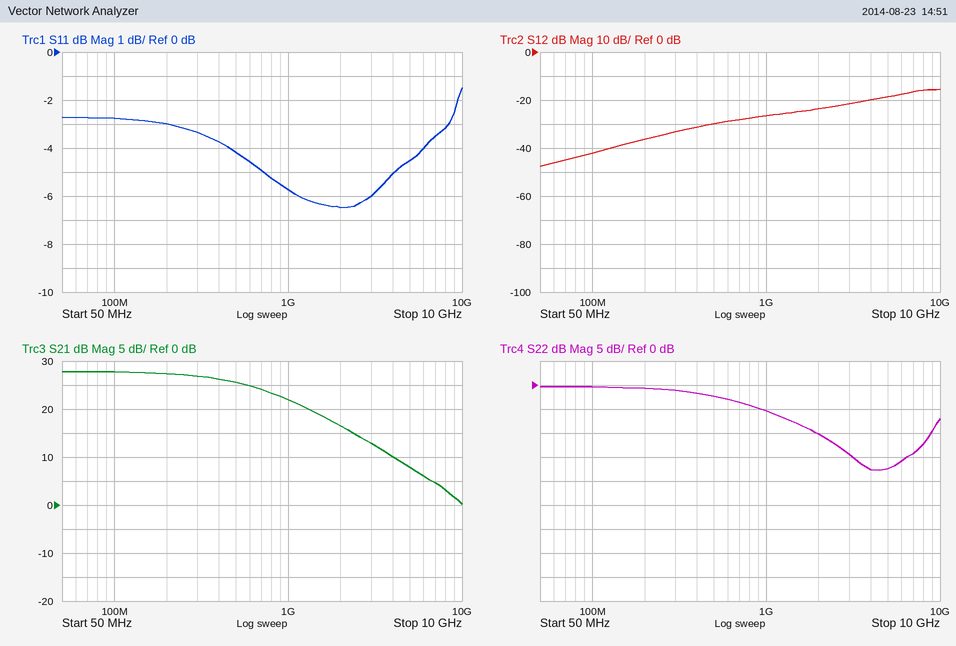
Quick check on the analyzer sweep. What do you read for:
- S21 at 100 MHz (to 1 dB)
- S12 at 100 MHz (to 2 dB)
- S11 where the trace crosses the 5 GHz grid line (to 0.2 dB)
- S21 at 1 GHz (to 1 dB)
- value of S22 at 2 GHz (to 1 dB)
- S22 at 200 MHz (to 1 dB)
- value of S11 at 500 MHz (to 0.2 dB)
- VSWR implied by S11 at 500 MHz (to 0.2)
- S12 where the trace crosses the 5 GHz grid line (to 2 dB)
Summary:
28 dB
-42 dB
-4.6 dB
22 dB
-10 dB
-1 dB
-4.2 dB
4.2
-18 dB
